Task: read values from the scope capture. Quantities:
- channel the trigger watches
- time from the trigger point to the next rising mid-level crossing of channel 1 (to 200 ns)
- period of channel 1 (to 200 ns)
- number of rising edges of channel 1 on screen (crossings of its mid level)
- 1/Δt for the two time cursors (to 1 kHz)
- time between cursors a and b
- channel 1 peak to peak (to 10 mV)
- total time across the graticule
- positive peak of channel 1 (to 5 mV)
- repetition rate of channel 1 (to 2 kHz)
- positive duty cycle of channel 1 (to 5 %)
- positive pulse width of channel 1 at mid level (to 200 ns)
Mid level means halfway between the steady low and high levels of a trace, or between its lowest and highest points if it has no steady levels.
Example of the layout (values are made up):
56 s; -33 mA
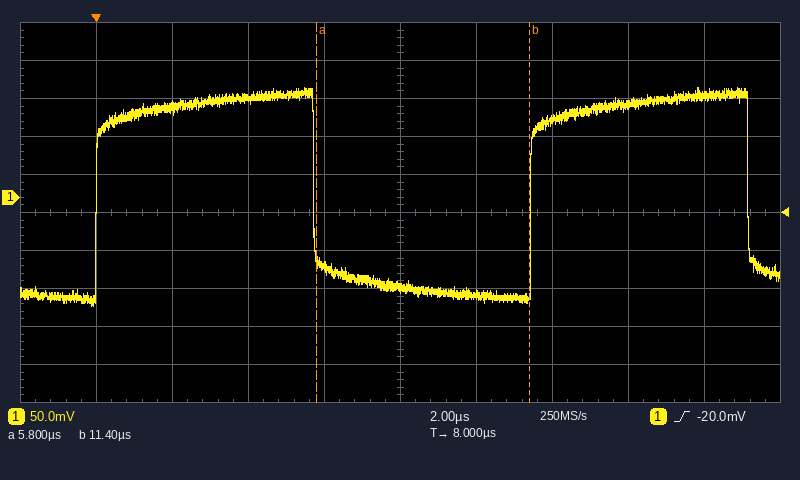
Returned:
channel 1; 11.4 µs; 11.4 µs; 2; 179 kHz; 5.6 µs; 290 mV; 20 µs; 145 mV; 88 kHz; 50 %; 5.8 µs
